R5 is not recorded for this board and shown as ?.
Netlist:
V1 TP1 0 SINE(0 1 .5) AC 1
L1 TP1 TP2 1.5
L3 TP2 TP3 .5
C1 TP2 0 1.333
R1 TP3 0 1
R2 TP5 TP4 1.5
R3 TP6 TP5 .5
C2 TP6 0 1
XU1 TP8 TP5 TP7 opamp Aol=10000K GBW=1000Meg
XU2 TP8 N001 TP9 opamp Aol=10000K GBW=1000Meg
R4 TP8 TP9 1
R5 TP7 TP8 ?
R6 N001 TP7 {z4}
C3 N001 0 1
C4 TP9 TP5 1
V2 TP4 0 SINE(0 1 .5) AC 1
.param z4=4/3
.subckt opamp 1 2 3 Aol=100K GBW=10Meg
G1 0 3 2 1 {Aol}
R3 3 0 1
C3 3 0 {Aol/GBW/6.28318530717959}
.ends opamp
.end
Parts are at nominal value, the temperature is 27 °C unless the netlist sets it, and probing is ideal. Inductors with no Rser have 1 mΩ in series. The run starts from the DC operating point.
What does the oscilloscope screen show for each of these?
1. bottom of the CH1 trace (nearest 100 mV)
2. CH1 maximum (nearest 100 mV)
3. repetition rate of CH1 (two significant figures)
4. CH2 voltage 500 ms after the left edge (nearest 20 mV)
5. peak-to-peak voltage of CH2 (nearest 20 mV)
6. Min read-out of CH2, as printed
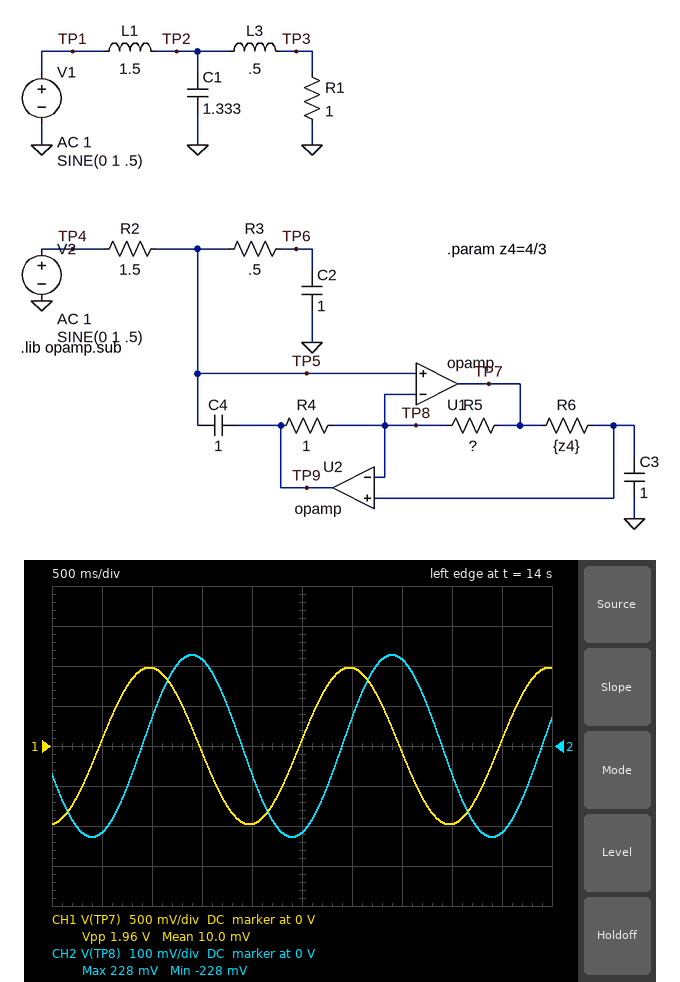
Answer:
-1.0 V
1.0 V
500 mHz
-220 mV
460 mV
-228 mV
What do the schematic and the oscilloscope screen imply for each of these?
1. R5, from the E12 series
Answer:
2.7 Ω
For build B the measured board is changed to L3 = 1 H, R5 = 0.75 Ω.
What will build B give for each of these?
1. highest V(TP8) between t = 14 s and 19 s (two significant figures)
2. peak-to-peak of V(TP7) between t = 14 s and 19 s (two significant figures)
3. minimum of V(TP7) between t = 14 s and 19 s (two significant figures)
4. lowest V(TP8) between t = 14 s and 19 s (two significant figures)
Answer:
43 mV
370 mV
-190 mV
-44 mV
